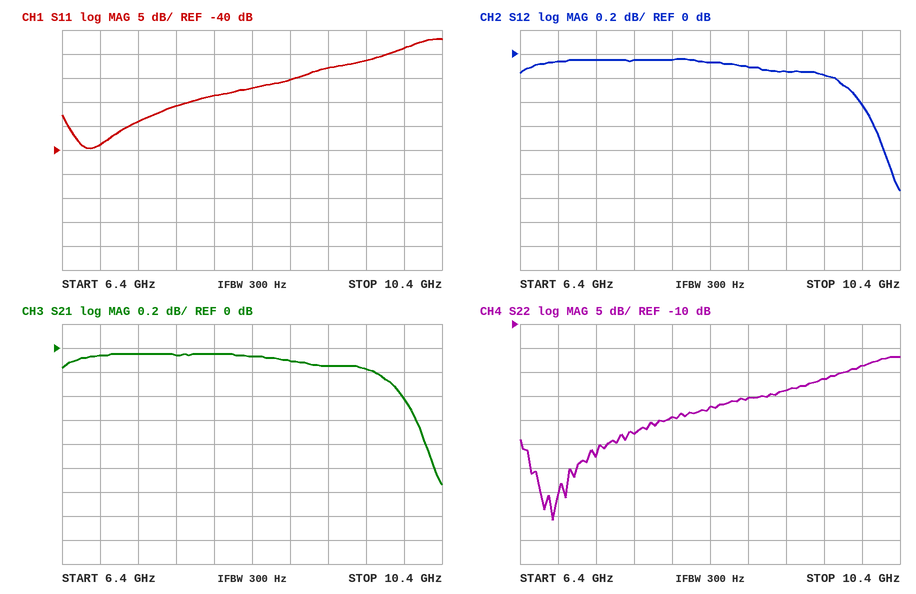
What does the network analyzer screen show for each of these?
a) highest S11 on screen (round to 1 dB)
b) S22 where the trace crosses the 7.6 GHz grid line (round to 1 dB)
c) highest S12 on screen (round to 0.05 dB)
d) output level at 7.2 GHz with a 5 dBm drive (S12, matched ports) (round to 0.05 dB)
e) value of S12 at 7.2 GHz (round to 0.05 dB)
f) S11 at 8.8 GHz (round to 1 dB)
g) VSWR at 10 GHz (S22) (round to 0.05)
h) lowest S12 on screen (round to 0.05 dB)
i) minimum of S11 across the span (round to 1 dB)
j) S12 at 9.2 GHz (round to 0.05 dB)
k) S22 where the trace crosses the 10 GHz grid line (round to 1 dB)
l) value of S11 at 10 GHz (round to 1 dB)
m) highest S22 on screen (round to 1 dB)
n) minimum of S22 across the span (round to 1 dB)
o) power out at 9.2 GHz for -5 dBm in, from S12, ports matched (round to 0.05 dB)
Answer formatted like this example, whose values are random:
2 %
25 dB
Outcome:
-17 dB
-33 dB
-0.05 dB
4.95 dBm
-0.05 dB
-25 dB
1.25
-1.15 dB
-40 dB
-0.15 dB
-19 dB
-19 dB
-17 dB
-51 dB
-5.15 dBm
